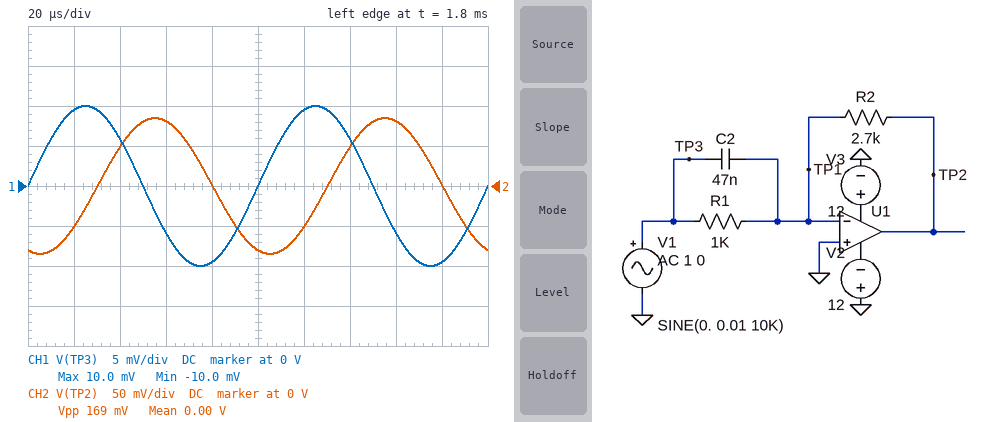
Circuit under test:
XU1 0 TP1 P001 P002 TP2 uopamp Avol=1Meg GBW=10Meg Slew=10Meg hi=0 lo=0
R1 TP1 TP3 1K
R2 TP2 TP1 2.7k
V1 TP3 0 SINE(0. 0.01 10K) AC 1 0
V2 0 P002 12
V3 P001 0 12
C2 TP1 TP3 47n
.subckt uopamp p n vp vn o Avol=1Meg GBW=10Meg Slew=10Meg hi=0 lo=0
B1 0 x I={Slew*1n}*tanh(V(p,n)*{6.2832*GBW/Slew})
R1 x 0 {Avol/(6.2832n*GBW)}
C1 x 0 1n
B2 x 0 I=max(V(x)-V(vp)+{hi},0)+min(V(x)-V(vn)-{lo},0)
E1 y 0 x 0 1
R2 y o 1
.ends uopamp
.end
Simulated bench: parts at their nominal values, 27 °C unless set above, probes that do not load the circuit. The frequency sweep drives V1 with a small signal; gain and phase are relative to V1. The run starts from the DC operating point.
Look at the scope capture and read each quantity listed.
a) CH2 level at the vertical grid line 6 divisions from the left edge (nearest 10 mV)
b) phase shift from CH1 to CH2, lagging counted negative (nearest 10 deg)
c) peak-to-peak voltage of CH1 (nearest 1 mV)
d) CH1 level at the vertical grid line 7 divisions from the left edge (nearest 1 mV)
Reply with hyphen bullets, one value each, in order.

- -50 mV
- -110 deg
- 20 mV
- 6 mV
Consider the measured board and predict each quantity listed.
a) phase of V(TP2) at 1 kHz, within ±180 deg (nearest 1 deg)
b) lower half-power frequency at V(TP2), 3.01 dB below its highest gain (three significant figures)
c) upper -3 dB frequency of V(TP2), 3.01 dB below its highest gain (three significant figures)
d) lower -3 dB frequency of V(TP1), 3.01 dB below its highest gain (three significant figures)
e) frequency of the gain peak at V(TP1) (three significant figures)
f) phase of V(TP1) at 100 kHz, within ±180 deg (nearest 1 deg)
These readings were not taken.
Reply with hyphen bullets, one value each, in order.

- -164 deg
- 110 kHz
- 114 kHz
- 110 kHz
- 112 kHz
- 168 deg
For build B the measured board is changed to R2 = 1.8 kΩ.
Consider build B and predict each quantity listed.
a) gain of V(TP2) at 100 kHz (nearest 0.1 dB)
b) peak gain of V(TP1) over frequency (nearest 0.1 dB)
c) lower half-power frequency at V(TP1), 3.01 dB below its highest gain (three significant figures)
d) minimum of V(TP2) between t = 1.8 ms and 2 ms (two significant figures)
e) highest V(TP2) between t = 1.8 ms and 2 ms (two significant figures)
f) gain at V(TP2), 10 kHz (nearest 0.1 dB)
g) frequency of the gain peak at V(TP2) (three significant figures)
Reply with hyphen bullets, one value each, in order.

- 41.1 dB
- 28.3 dB
- 135 kHz
- -56 mV
- 56 mV
- 15.0 dB
- 137 kHz
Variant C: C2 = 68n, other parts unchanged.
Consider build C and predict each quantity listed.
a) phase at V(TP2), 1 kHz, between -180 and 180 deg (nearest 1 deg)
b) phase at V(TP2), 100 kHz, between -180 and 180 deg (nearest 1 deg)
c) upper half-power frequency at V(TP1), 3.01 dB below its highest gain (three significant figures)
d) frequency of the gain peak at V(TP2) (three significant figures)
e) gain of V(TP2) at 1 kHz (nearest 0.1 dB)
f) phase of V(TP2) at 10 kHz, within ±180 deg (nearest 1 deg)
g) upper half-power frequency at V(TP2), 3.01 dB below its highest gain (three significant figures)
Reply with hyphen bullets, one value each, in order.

- -157 deg
- 102 deg
- 94.8 kHz
- 93.1 kHz
- 9.4 dB
- -103 deg
- 94.7 kHz
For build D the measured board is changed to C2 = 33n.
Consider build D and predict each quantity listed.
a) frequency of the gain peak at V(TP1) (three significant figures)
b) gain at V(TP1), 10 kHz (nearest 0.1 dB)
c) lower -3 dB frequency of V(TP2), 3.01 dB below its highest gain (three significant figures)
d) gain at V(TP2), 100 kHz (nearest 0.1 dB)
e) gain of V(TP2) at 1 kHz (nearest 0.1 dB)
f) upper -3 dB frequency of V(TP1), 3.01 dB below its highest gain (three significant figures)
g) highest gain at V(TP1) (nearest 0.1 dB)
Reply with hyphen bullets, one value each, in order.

- 134 kHz
- -44.1 dB
- 130 kHz
- 42.1 dB
- 8.8 dB
- 137 kHz
- 26.1 dB
